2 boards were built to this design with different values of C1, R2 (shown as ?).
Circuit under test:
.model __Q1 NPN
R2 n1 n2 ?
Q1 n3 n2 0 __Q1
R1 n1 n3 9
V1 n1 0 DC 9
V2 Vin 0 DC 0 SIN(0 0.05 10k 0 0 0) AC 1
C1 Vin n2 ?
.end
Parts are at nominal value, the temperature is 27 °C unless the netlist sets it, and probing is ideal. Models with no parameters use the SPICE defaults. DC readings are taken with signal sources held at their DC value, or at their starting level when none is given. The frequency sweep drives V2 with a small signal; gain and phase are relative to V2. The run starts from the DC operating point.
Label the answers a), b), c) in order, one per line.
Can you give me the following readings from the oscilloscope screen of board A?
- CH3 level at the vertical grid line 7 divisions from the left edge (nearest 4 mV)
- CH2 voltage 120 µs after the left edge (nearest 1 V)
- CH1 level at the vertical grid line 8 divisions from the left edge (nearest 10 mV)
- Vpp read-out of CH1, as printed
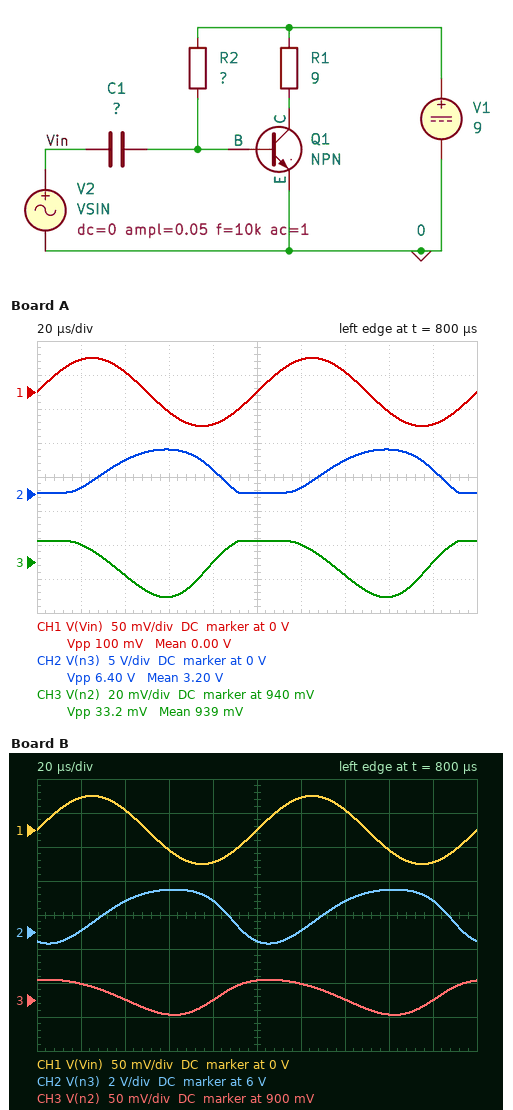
a) 932 mV
b) 1 V
c) -30 mV
d) 100 mV
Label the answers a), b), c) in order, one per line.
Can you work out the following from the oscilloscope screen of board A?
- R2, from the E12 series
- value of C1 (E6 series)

a) 1.2 kΩ
b) 1.5 µF
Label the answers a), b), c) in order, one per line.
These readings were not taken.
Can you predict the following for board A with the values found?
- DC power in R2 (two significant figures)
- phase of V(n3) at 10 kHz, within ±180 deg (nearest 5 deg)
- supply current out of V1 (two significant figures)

a) 54 mW
b) -110 deg
c) 680 mA
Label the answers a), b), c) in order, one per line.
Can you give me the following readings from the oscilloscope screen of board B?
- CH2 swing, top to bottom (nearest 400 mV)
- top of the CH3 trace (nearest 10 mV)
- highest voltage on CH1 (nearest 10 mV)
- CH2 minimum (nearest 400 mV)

a) 3.2 V
b) 930 mV
c) 50 mV
d) 5.2 V
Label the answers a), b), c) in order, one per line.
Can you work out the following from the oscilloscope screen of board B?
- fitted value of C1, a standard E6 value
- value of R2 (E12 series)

a) 680 nF
b) 3.9 kΩ
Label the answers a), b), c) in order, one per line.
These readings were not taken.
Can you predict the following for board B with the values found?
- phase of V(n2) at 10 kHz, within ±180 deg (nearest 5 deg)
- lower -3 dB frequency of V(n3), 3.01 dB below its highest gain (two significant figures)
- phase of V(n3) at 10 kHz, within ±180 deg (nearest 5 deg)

a) 60 deg
b) 19 kHz
c) -120 deg
